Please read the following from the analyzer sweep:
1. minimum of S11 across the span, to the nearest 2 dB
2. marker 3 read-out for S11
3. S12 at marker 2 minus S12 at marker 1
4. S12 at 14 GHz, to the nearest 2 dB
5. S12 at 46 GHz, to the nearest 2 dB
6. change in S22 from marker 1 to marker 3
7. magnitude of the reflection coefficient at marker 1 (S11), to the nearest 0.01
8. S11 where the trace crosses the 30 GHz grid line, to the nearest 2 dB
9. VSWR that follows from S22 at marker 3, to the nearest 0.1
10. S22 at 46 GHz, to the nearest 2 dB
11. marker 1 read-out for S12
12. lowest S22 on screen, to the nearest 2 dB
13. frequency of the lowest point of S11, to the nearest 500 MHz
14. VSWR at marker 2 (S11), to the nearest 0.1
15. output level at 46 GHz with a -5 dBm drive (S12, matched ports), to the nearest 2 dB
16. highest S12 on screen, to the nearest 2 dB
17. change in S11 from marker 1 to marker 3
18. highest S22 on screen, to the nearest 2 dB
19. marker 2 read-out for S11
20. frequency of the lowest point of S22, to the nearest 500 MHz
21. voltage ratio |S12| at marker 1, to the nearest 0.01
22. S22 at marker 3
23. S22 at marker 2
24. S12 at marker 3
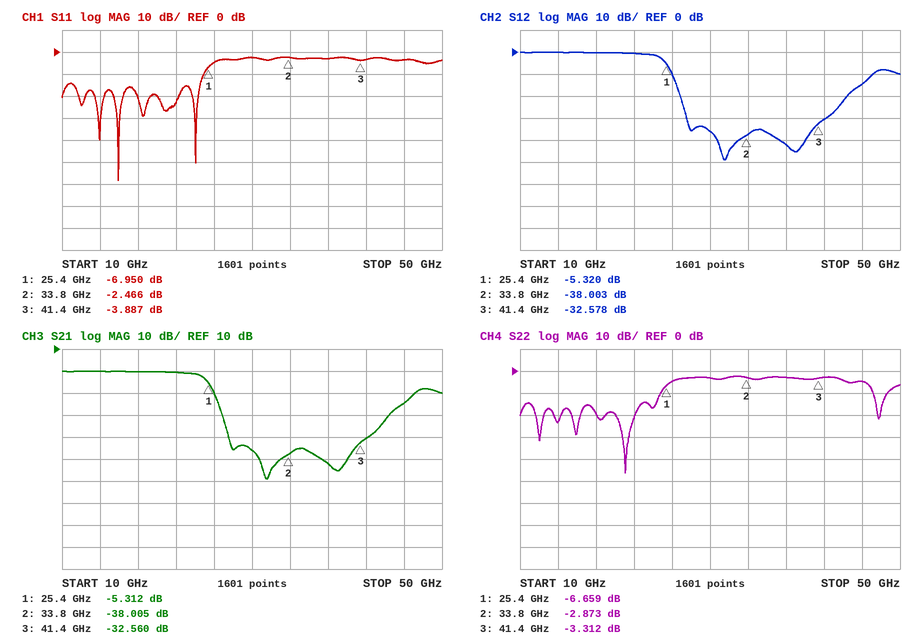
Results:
-58 dB
-3.887 dB
-32.683 dB
0 dB
-14 dB
3.347 dB
0.45
-2 dB
5.3
-4 dB
-5.320 dB
-46 dB
16.0 GHz
7.1
-20 dBm
0 dB
3.063 dB
-2 dB
-2.466 dB
21.0 GHz
0.54
-3.312 dB
-2.873 dB
-32.578 dB
